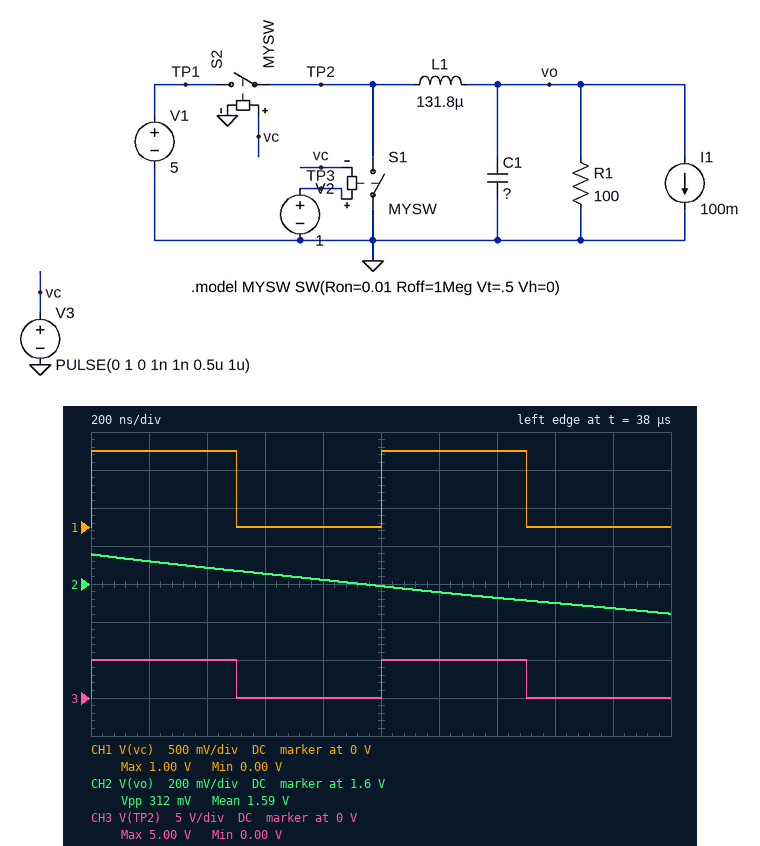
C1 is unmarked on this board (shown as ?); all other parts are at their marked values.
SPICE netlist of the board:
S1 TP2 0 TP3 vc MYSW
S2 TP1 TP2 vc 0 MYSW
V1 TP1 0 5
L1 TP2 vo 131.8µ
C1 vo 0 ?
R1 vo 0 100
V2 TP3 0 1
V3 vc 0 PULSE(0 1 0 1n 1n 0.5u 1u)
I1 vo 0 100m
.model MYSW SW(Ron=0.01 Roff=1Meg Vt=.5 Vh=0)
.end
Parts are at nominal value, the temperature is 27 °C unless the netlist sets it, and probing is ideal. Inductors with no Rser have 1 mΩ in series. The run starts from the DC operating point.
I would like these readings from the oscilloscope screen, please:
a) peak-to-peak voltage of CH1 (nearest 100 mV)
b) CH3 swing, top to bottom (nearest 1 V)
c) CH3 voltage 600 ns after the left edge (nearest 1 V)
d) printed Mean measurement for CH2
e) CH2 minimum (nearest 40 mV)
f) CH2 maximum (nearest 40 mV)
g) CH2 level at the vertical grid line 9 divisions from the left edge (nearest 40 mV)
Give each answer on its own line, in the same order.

1.0 V
5 V
0 V
1.59 V
1.44 V
1.76 V
1.48 V
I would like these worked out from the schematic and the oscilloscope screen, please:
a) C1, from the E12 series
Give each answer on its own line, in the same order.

390 nF
